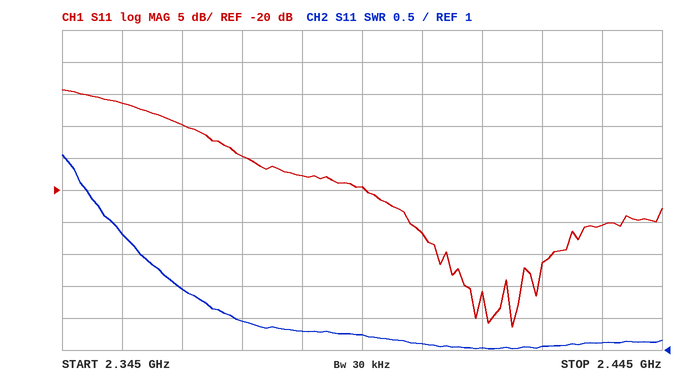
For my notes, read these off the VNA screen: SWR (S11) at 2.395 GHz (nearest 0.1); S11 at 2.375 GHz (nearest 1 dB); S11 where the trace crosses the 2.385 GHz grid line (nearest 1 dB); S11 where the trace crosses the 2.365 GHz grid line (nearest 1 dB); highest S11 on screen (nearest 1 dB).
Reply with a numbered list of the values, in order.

1. 1.2
2. -15 dB
3. -18 dB
4. -10 dB
5. -4 dB
